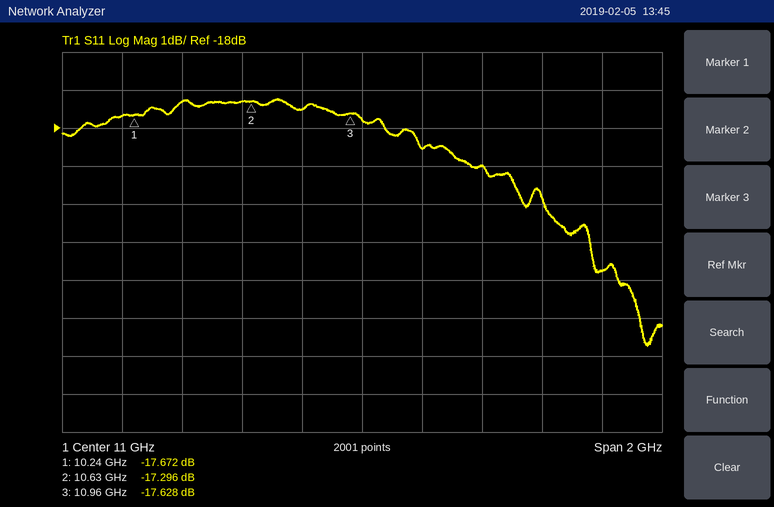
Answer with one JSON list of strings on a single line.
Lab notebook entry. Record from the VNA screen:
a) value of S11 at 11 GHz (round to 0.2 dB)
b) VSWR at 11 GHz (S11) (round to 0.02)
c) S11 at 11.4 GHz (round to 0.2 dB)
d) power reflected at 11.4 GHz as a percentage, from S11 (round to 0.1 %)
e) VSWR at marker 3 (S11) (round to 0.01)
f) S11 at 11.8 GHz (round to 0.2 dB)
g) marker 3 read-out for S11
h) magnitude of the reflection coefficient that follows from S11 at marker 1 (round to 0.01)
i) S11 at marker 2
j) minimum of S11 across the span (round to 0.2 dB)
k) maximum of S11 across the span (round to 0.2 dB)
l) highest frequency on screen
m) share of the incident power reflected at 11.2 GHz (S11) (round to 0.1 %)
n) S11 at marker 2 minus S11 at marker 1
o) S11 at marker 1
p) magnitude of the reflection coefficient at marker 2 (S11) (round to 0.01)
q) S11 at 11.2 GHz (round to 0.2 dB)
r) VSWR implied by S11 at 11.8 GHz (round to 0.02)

["-17.8 dB", "1.30", "-19.0 dB", "1.3 %", "1.30", "-21.8 dB", "-17.628 dB", "0.13", "-17.296 dB", "-23.8 dB", "-17.2 dB", "12 GHz", "1.4 %", "0.376 dB", "-17.672 dB", "0.14", "-18.6 dB", "1.18"]
